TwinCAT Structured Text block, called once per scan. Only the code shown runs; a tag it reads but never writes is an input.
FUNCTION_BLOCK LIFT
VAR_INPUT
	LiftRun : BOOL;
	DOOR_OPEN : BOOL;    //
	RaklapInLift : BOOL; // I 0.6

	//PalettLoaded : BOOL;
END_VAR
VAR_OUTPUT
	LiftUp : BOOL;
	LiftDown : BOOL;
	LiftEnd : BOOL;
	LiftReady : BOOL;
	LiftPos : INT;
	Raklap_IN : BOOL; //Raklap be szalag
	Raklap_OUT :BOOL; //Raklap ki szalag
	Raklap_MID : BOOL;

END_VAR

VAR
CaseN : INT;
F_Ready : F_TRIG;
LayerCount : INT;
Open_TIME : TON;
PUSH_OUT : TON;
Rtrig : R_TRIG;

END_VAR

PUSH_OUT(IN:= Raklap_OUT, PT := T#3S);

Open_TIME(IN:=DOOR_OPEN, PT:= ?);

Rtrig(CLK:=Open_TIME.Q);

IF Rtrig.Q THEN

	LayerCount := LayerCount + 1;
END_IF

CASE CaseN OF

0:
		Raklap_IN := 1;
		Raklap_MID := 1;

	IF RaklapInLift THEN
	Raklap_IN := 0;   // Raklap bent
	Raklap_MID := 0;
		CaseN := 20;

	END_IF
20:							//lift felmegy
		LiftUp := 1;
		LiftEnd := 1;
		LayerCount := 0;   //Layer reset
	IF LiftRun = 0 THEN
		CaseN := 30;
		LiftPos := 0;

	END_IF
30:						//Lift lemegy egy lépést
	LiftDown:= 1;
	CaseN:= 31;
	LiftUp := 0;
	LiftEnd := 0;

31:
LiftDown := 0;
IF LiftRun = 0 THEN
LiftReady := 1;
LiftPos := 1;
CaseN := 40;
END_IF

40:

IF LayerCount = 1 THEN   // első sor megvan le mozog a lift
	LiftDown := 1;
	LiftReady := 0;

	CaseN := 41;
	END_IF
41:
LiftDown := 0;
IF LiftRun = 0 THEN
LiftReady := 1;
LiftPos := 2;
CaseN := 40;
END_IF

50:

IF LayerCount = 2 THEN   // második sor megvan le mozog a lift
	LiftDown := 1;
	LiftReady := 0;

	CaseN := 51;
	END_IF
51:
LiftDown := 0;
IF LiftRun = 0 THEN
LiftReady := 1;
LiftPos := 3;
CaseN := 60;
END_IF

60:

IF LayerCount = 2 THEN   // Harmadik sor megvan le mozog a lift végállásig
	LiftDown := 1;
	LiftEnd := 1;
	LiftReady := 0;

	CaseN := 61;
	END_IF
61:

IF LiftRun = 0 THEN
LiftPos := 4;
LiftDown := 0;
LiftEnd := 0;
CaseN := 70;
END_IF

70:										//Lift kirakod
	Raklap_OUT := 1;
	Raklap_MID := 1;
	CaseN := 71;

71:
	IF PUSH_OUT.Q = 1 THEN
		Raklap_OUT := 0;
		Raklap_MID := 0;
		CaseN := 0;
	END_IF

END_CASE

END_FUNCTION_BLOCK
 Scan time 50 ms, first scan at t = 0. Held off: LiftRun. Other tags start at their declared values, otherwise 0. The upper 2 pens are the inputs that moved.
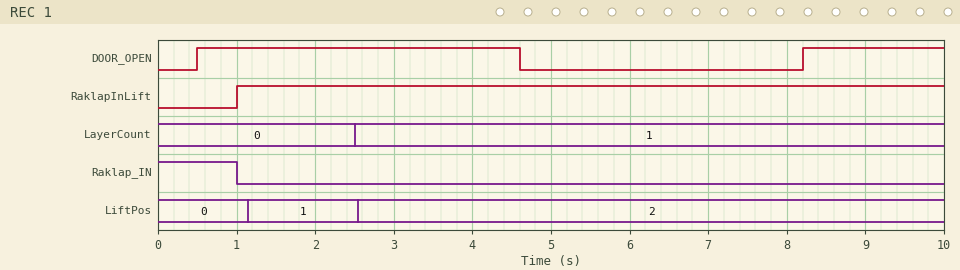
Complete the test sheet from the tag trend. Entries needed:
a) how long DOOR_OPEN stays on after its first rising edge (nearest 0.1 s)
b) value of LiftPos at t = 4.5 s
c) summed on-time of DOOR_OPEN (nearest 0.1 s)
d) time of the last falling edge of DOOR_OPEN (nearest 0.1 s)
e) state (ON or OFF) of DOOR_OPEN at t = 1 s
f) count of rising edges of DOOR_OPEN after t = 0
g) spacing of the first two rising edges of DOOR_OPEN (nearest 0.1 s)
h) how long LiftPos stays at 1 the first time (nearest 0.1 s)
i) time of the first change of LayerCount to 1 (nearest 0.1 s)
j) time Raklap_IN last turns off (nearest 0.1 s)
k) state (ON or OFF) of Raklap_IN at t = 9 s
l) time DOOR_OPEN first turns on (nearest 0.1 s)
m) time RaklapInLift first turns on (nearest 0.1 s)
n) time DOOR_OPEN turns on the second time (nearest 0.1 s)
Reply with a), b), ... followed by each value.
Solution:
a) 4.1 s
b) 2
c) 5.9 s
d) 4.6 s
e) ON
f) 2
g) 7.7 s
h) 1.4 s
i) 2.5 s
j) 1.0 s
k) OFF
l) 0.5 s
m) 1.0 s
n) 8.2 s
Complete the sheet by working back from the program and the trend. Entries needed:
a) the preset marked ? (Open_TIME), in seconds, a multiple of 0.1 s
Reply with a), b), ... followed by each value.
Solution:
a) 2.0 s
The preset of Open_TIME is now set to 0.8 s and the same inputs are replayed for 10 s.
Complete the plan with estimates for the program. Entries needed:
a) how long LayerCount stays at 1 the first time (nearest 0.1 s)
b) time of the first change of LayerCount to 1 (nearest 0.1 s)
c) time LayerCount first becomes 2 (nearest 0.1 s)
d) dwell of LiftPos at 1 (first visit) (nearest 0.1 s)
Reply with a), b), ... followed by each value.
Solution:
a) 7.7 s
b) 1.3 s
c) 9.0 s
d) 0.2 s
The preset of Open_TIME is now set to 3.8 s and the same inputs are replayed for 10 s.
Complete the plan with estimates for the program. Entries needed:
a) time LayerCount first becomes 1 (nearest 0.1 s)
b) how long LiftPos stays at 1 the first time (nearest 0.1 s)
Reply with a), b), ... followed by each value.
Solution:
a) 4.3 s
b) 3.2 s
